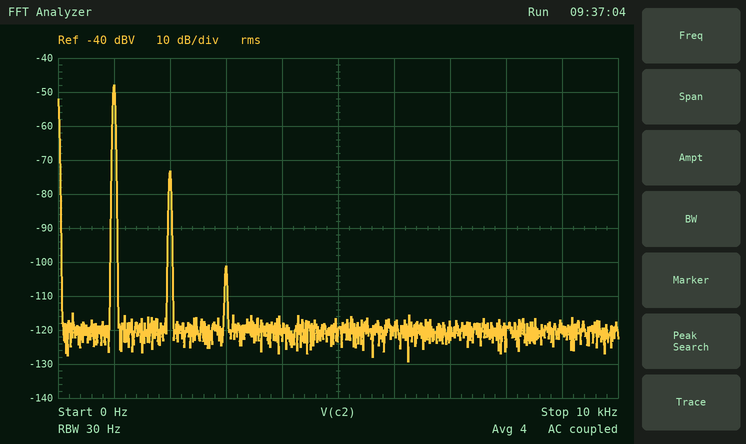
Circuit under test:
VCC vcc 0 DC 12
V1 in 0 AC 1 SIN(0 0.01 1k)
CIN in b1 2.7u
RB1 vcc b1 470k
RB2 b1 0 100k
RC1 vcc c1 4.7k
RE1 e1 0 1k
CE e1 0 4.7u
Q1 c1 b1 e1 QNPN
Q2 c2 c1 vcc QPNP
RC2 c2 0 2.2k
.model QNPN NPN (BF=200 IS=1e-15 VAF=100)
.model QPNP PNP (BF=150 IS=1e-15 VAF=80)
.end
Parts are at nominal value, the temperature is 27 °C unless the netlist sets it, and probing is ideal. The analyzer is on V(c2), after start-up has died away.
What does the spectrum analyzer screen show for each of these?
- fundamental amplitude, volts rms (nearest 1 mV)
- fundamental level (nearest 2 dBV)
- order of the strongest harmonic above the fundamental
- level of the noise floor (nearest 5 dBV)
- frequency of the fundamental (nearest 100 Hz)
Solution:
4 mV
-48 dBV
2
-120 dBV
1.0 kHz
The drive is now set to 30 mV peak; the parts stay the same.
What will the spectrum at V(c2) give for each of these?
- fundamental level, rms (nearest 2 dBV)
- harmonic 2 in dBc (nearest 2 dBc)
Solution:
-38 dBV
-16 dBc
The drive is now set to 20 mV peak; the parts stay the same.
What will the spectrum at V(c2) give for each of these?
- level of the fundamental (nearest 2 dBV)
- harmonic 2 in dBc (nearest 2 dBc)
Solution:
-42 dBV
-20 dBc
